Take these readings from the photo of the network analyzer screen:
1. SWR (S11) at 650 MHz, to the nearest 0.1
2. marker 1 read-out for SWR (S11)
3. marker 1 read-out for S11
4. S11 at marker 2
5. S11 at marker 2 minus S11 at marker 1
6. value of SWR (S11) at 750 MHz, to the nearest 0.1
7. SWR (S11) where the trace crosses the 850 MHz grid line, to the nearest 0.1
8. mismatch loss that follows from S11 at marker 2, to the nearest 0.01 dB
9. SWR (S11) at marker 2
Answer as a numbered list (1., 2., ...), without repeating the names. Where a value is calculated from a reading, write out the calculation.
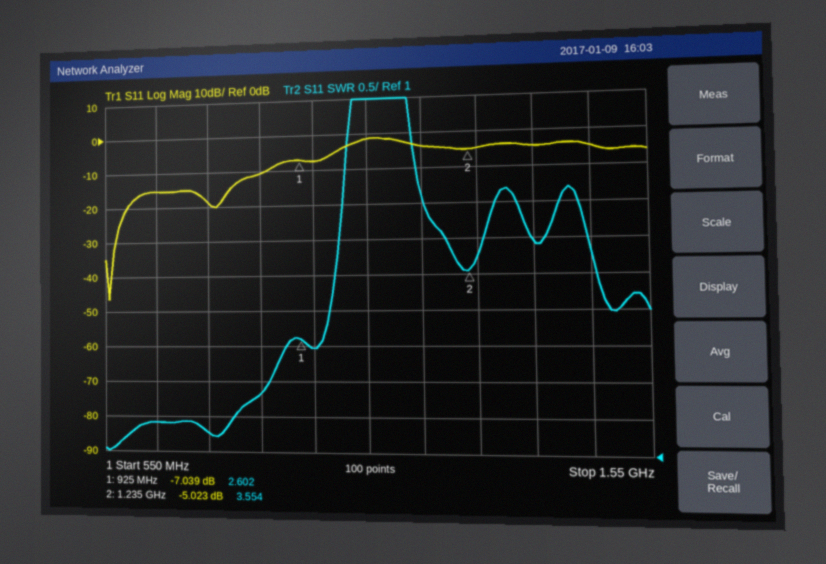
1. 1.4
2. 2.602
3. -7.039 dB
4. -5.023 dB
5. -5.023 − (-7.039) = 2.016 dB
6. 1.3
7. 1.8
8. −10 log10(1 − 10^(-5.023/10)) ≈ 1.64 dB
9. 3.554
